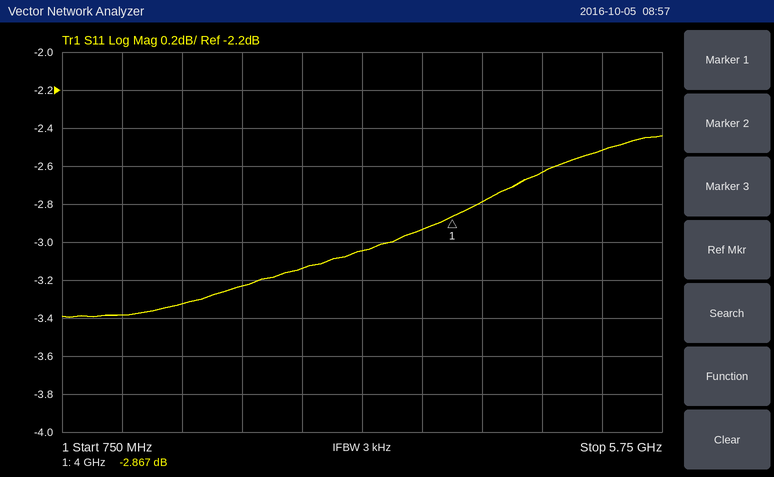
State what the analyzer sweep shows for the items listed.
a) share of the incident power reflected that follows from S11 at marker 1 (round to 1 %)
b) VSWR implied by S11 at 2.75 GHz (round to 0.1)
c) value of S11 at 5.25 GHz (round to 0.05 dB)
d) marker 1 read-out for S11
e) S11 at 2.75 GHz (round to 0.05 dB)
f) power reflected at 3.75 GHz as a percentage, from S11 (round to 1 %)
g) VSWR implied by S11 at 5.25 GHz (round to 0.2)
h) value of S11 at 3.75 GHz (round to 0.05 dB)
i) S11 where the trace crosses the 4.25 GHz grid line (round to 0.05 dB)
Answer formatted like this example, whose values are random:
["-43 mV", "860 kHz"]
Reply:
["52 %", "5.6", "-2.50 dB", "-2.867 dB", "-3.15 dB", "51 %", "7.0", "-2.95 dB", "-2.80 dB"]
